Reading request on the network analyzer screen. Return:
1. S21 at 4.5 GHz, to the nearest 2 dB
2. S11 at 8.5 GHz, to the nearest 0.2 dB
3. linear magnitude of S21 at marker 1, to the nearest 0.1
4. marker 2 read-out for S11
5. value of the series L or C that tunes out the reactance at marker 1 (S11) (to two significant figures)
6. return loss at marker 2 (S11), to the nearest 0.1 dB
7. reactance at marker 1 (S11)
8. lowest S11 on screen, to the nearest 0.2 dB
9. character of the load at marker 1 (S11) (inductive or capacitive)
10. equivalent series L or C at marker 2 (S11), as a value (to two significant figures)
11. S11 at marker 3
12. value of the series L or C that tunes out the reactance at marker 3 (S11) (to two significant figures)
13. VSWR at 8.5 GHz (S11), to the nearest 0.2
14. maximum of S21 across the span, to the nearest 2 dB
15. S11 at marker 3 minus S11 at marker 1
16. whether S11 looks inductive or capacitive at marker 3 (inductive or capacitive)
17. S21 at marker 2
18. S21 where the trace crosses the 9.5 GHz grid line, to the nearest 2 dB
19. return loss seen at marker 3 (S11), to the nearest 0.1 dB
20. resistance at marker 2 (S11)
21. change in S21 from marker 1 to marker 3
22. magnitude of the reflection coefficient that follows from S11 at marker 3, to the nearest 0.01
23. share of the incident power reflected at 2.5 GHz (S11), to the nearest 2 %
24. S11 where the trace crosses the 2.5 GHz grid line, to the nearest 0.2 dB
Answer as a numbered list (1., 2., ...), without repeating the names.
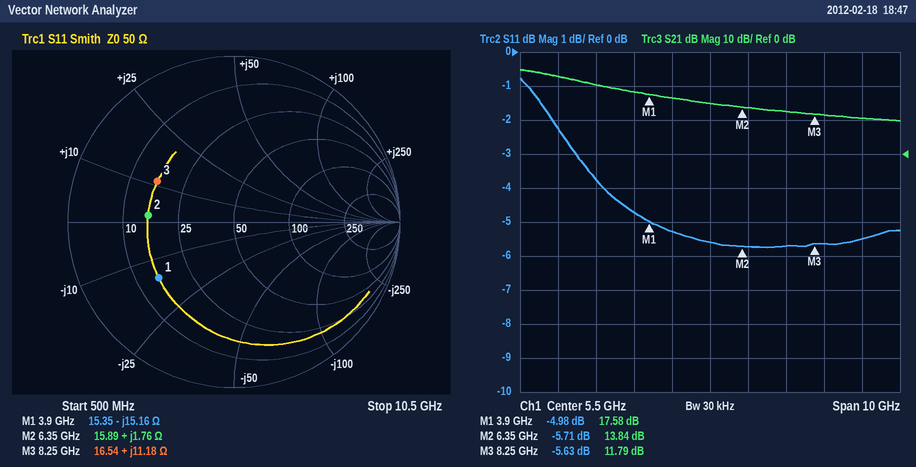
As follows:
1. 16 dB
2. -5.6 dB
3. 7.6
4. -5.71 dB
5. 620 pH
6. 5.7 dB
7. -15.16 Ω
8. -5.8 dB
9. capacitive
10. 44 pH
11. -5.63 dB
12. 1.7 pF
13. 3.2
14. 24 dB
15. -0.65 dB
16. inductive
17. 13.84 dB
18. 10 dB
19. 5.6 dB
20. 15.89 Ω
21. -5.79 dB
22. 0.52
23. 42 %
24. -3.8 dB
